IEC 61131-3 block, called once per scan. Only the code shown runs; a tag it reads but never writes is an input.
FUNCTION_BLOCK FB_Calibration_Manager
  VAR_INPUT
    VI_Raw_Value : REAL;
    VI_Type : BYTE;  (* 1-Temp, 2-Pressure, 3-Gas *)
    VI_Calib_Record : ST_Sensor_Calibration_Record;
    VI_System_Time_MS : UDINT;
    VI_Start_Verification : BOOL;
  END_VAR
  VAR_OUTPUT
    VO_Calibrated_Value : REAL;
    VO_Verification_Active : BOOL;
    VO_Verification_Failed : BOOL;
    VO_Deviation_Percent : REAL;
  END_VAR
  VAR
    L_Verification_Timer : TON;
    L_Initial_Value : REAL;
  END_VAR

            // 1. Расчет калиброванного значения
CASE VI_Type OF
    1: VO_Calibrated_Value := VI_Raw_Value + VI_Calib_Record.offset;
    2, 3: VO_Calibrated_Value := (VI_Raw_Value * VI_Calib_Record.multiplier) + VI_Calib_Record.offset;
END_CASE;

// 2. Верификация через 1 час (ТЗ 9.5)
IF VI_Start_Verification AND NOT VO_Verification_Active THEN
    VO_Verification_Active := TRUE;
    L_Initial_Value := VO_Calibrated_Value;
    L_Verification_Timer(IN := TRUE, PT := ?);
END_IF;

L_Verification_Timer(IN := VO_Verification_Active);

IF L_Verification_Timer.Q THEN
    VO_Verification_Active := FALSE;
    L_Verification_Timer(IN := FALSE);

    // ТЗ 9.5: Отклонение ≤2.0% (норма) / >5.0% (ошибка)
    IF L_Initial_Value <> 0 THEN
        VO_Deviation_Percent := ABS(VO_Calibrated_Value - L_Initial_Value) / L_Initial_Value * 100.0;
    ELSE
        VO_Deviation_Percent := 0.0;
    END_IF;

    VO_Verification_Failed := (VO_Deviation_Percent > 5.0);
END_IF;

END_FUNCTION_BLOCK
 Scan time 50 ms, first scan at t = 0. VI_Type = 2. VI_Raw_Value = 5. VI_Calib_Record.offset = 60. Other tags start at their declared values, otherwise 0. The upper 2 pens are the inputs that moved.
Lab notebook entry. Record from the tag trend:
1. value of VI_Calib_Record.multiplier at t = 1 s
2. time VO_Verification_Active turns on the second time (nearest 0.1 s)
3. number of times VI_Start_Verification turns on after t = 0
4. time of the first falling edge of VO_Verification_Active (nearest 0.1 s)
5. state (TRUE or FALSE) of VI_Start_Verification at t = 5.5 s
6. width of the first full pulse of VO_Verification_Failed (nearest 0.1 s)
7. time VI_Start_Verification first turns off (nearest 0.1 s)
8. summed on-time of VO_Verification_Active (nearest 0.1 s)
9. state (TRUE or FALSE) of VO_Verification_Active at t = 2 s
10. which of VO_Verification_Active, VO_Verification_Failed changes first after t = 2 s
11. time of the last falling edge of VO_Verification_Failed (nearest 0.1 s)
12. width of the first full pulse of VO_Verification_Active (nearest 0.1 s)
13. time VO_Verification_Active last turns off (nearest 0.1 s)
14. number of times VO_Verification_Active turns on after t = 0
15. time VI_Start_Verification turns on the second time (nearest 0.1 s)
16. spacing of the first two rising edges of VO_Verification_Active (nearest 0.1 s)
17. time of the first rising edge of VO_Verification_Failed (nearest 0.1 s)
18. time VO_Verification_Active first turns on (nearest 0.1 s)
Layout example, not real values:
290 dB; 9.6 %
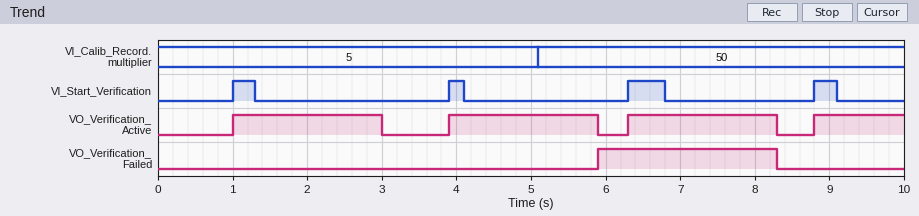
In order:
5; 3.9 s; 4; 3.0 s; FALSE; 2.4 s; 1.3 s; 7.2 s; TRUE; VO_Verification_Active; 8.3 s; 2.0 s; 8.3 s; 4; 3.9 s; 2.9 s; 5.9 s; 1.0 s
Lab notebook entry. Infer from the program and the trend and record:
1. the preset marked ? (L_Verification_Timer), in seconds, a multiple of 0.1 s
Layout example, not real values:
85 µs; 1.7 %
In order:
2.0 s
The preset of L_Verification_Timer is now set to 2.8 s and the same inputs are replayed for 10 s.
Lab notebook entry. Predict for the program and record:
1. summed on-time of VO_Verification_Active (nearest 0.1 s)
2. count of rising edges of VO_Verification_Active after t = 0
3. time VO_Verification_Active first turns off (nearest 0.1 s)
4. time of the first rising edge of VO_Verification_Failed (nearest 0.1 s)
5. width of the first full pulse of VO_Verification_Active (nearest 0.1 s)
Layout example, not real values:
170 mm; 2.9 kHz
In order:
8.4 s; 3; 3.8 s; 6.7 s; 2.8 s
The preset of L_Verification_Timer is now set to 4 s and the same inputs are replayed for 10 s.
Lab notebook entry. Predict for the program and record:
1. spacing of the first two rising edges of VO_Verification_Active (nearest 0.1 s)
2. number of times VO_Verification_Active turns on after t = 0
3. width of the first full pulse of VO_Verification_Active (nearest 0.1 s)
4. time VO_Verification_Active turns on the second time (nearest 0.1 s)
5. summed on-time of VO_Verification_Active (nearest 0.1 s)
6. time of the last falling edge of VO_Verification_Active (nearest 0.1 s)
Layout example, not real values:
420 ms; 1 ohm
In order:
5.3 s; 2; 4.0 s; 6.3 s; 7.7 s; 5.0 s
